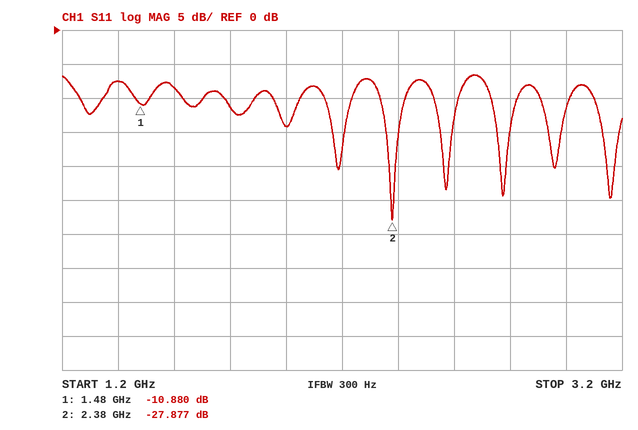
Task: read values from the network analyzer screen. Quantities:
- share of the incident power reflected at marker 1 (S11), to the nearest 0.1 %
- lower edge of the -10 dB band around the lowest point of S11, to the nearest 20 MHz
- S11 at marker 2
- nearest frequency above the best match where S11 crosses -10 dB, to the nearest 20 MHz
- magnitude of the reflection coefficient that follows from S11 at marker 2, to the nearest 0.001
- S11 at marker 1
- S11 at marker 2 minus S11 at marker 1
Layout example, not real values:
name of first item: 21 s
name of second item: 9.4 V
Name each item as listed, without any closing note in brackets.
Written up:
share of the incident power reflected at marker 1 (S11), to the nearest 0.1 %: 8.2 %
lower edge of the -10 dB band around the lowest point of S11, to the nearest 20 MHz: 2.34 GHz
S11 at marker 2: -27.877 dB
nearest frequency above the best match where S11 crosses -10 dB, to the nearest 20 MHz: 2.42 GHz
magnitude of the reflection coefficient that follows from S11 at marker 2, to the nearest 0.001: 0.040
S11 at marker 1: -10.880 dB
S11 at marker 2 minus S11 at marker 1: -16.997 dB
